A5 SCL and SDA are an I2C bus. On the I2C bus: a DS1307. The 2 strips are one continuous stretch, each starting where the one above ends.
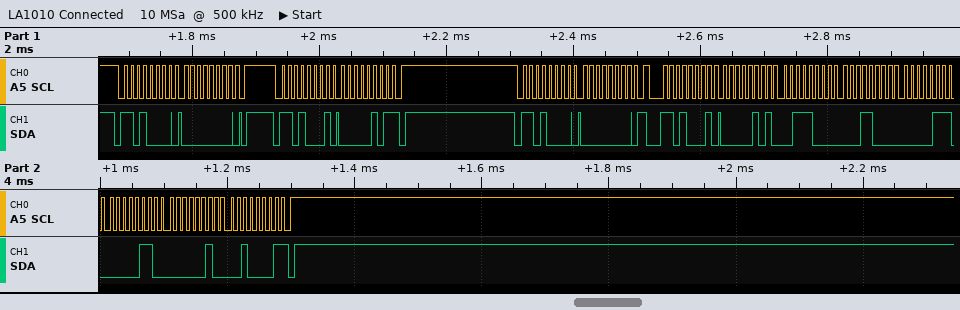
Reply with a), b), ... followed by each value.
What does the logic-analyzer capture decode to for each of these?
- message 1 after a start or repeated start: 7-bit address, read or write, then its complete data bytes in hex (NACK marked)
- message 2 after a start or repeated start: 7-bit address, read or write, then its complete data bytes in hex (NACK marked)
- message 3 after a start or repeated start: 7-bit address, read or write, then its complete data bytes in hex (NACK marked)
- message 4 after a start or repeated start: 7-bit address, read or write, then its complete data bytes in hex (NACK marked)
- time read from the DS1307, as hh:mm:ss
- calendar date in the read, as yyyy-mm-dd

a) 0x68 write: 00
b) 0x68 read: 05 NACK
c) 0x68 write: 00
d) 0x68 read: 05 38 18 07 06 02 21 NACK
e) 18:38:05
f) 2021-02-06
